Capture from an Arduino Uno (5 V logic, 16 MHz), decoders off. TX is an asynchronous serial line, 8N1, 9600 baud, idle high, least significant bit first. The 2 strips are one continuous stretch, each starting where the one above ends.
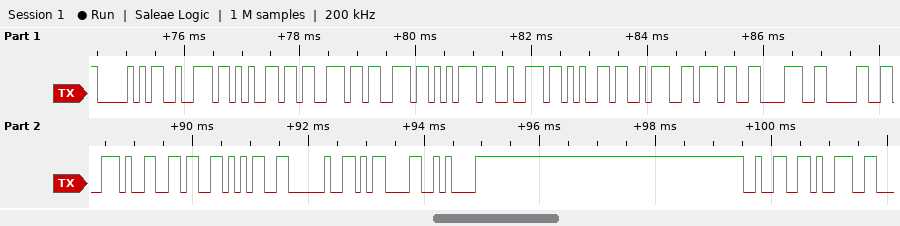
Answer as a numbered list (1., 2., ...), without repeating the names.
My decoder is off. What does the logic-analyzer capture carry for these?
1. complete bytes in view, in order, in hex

1. 50 72 65 73 73 75 72 65 3A 37 38 30 2E 36 35 20 0D 0A 32 39
